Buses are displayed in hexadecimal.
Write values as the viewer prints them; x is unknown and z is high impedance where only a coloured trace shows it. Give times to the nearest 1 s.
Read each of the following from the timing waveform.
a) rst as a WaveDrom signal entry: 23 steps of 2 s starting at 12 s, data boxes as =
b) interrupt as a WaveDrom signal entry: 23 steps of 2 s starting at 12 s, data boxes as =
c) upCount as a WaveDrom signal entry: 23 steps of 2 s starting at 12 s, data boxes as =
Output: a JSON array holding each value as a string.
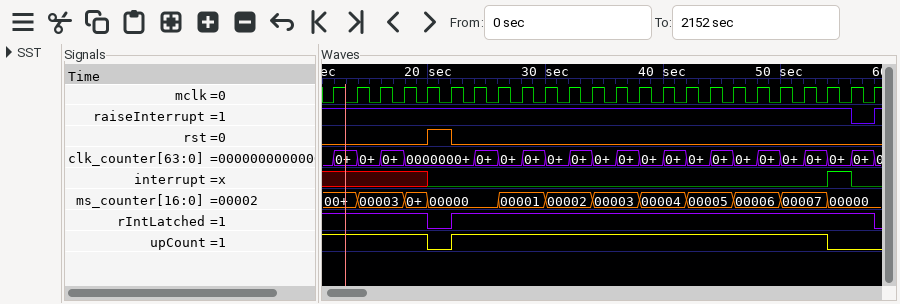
["{name: 'rst', wave: '0...10.................'}", "{name: 'interrupt', wave: 'x...0................10'}", "{name: 'upCount', wave: '1...01...............0.'}"]
